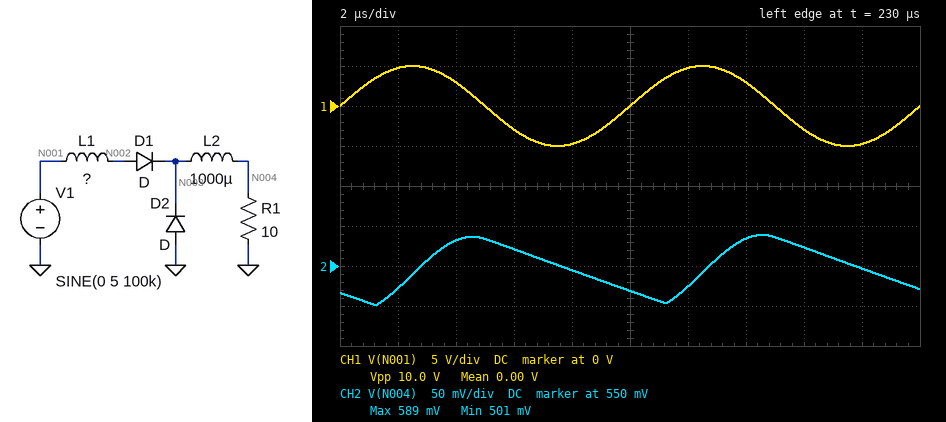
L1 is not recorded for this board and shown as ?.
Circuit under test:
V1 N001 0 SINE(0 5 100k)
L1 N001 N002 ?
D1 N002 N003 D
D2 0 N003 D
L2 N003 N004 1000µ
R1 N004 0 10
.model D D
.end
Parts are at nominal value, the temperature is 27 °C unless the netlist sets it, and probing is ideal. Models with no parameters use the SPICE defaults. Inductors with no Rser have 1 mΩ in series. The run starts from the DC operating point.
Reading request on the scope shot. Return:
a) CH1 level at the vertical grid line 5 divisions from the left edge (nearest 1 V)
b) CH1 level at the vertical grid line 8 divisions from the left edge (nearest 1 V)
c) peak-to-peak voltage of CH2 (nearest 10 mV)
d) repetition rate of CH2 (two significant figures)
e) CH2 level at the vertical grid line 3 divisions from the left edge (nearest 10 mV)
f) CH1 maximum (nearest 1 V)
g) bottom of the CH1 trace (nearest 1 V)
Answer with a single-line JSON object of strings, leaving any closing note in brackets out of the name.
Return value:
{"CH1 level at the vertical grid line 5 divisions from the left edge": "0 V", "CH1 level at the vertical grid line 8 divisions from the left edge": "-3 V", "peak-to-peak voltage of CH2": "90 mV", "repetition rate of CH2": "100 kHz", "CH2 level at the vertical grid line 3 divisions from the left edge": "570 mV", "CH1 maximum": "5 V", "bottom of the CH1 trace": "-5 V"}
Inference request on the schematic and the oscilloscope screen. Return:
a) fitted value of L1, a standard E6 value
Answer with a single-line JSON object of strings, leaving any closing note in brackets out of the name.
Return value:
{"fitted value of L1, a standard E6 value": "47 µH"}
